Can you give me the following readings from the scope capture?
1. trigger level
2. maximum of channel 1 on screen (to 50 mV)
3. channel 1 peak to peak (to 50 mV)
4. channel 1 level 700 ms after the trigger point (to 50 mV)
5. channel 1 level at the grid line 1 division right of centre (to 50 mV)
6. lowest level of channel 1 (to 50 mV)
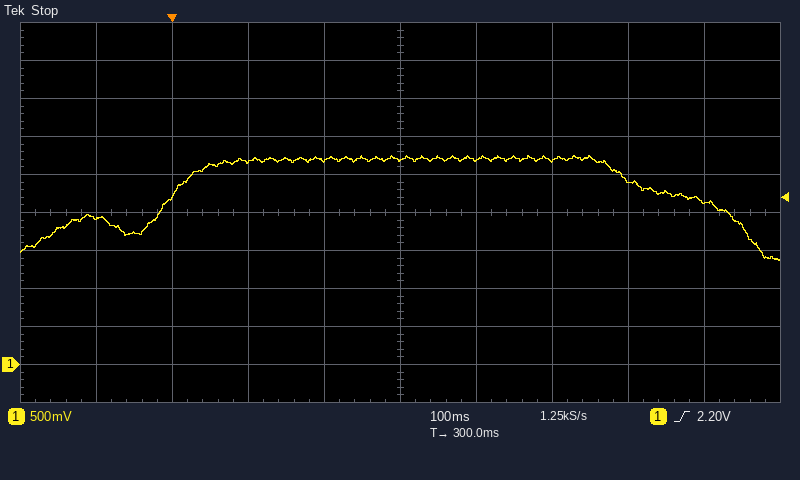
2.20 V
2.75 V
1.40 V
2.15 V
2.70 V
1.35 V
